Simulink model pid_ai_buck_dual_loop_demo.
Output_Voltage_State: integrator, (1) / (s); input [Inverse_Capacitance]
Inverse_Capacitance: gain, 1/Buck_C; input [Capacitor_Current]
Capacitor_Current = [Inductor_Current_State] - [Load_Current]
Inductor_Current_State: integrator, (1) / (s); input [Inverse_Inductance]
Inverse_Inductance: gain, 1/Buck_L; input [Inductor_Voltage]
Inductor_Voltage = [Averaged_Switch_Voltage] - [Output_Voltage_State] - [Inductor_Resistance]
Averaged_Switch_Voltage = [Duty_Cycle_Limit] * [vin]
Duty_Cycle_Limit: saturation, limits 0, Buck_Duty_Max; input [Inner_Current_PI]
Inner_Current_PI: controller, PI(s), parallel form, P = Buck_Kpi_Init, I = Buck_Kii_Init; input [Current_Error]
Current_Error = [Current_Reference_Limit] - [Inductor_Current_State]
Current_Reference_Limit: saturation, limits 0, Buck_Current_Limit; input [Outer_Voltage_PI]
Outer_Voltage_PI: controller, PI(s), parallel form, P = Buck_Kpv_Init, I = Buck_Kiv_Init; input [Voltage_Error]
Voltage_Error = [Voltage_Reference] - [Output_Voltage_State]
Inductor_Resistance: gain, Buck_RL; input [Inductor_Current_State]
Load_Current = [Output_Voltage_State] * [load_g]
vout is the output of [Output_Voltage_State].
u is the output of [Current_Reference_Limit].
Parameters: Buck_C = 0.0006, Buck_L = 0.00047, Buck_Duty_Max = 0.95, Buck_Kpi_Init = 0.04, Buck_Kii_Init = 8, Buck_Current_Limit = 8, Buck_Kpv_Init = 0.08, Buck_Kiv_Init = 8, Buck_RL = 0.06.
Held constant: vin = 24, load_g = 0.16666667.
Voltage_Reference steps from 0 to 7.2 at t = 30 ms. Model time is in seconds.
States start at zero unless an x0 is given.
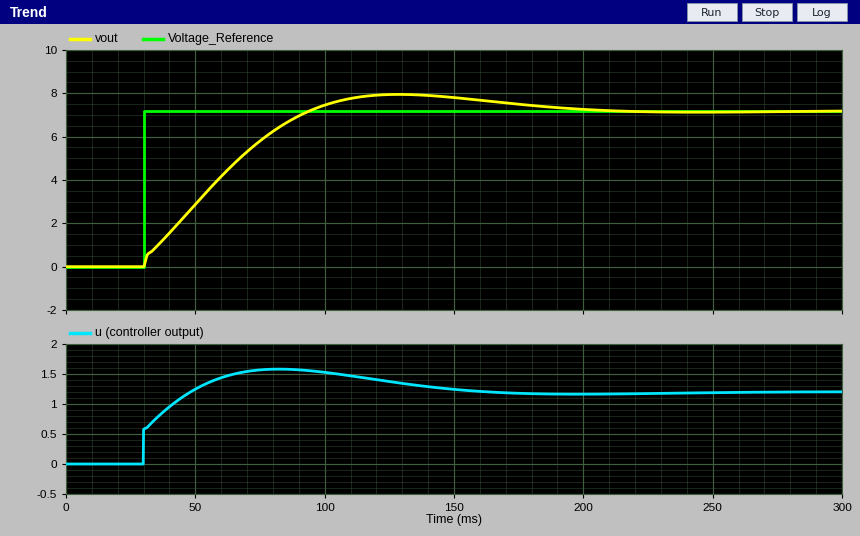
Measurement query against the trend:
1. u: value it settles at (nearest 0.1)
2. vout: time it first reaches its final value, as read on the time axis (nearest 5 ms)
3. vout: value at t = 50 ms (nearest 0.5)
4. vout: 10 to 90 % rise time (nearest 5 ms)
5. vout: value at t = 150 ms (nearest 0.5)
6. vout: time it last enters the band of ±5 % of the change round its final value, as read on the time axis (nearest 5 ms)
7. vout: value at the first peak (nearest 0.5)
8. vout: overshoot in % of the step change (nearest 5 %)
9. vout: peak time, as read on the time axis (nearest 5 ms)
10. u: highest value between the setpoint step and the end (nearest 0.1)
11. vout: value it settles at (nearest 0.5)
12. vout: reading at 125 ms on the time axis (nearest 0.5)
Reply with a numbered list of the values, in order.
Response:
1. 1.2
2. 95 ms
3. 3.0
4. 50 ms
5. 8.0
6. 170 ms
7. 8.0
8. 10 %
9. 130 ms
10. 1.6
11. 7.0
12. 8.0
